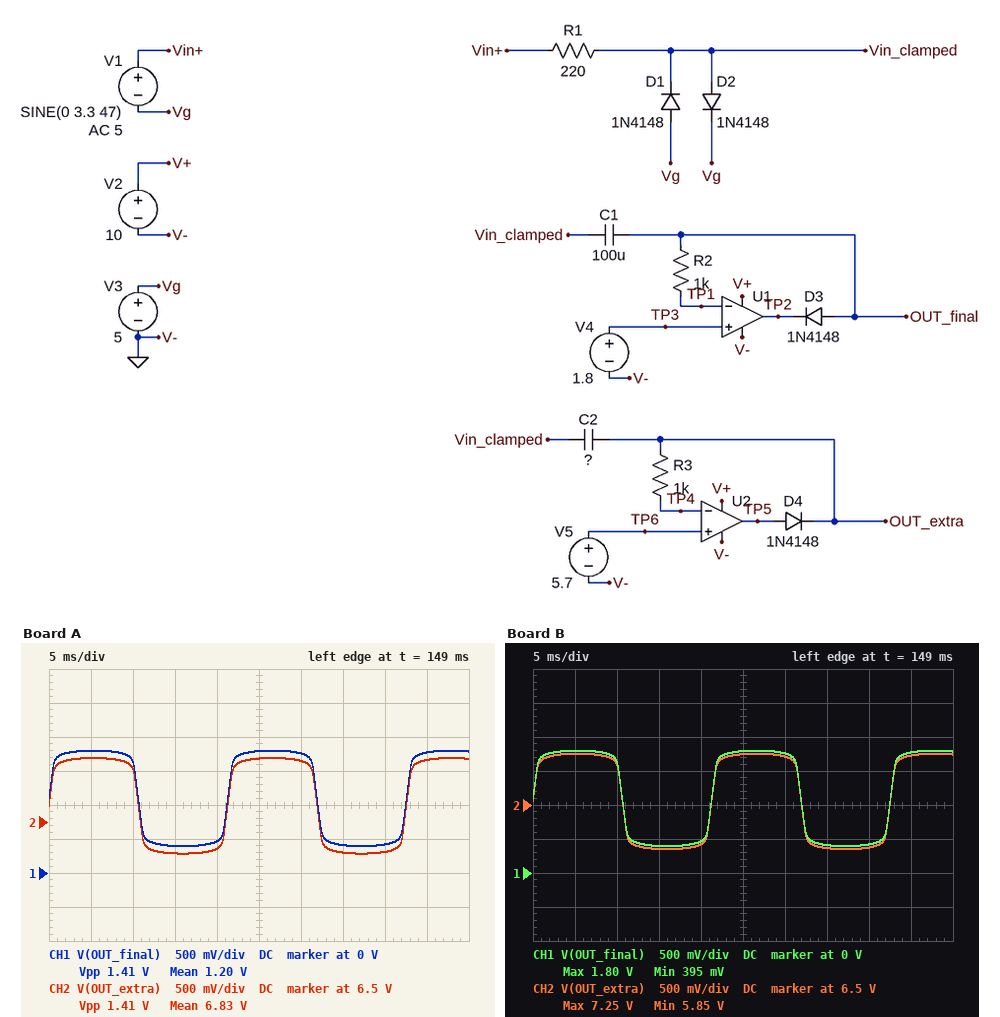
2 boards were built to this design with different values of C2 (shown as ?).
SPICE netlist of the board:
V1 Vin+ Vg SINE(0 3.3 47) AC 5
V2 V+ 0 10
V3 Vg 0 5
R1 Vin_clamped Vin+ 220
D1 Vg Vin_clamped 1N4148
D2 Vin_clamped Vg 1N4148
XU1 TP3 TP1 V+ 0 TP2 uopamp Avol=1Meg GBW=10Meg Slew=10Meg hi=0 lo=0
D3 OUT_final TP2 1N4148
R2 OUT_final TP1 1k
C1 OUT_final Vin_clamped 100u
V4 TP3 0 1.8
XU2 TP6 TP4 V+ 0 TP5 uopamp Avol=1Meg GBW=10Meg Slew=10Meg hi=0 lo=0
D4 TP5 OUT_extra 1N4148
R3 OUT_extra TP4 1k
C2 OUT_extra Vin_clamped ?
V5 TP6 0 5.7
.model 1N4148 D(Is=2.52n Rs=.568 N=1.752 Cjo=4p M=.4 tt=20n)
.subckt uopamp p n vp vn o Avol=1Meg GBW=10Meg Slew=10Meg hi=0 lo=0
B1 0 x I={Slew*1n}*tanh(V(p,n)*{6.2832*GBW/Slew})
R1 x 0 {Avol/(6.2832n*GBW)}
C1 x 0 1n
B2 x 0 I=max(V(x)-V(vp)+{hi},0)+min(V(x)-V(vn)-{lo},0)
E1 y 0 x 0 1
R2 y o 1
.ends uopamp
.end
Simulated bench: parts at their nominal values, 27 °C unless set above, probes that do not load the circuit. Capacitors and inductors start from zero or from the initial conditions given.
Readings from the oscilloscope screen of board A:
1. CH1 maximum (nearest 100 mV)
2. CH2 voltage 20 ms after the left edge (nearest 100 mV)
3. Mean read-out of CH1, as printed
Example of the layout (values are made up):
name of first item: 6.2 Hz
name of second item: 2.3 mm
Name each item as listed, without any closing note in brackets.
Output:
CH1 maximum: 1.8 V
CH2 voltage 20 ms after the left edge: 6.1 V
Mean read-out of CH1, as printed: 1.20 V
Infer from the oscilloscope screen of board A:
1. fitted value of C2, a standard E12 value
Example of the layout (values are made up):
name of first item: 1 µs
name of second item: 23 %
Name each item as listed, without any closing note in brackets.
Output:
fitted value of C2, a standard E12 value: 120 µF
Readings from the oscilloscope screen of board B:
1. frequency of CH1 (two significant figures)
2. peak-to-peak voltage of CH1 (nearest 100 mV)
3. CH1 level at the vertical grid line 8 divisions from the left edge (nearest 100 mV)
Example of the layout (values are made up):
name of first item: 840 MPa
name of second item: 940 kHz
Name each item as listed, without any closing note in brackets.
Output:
frequency of CH1: 47 Hz
peak-to-peak voltage of CH1: 1.4 V
CH1 level at the vertical grid line 8 divisions from the left edge: 400 mV
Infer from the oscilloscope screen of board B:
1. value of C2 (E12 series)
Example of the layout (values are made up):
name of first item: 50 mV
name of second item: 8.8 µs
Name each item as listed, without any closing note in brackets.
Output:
value of C2: 150 µF
